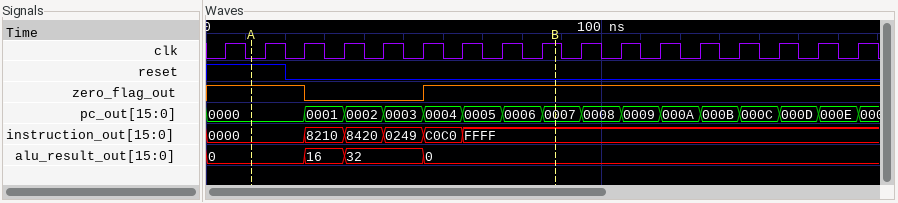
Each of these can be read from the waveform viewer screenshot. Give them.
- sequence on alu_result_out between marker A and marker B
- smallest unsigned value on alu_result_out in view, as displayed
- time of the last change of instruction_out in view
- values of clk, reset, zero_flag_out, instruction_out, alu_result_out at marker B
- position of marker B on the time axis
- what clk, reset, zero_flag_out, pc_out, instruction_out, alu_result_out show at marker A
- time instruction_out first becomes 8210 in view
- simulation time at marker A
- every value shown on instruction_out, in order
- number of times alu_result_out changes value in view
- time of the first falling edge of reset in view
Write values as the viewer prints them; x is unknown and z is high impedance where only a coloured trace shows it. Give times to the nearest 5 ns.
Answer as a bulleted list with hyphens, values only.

- 0, 16, 32, 0
- 0
- 65 ns
- clk=1, reset=0, zero_flag_out=1, instruction_out=FFFF, alu_result_out=0
- 90 ns
- clk=0, reset=1, zero_flag_out=1, pc_out=0000, instruction_out=0000, alu_result_out=0
- 25 ns
- 10 ns
- 0000, 8210, 8420, 0249, C0C0, FFFF
- 3
- 20 ns
